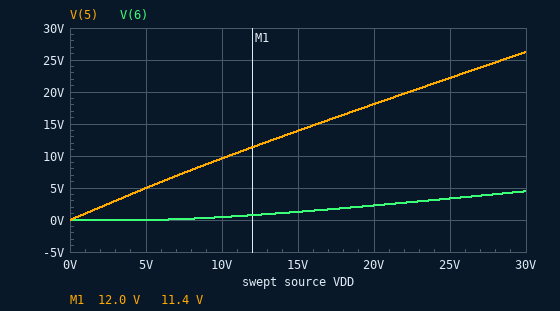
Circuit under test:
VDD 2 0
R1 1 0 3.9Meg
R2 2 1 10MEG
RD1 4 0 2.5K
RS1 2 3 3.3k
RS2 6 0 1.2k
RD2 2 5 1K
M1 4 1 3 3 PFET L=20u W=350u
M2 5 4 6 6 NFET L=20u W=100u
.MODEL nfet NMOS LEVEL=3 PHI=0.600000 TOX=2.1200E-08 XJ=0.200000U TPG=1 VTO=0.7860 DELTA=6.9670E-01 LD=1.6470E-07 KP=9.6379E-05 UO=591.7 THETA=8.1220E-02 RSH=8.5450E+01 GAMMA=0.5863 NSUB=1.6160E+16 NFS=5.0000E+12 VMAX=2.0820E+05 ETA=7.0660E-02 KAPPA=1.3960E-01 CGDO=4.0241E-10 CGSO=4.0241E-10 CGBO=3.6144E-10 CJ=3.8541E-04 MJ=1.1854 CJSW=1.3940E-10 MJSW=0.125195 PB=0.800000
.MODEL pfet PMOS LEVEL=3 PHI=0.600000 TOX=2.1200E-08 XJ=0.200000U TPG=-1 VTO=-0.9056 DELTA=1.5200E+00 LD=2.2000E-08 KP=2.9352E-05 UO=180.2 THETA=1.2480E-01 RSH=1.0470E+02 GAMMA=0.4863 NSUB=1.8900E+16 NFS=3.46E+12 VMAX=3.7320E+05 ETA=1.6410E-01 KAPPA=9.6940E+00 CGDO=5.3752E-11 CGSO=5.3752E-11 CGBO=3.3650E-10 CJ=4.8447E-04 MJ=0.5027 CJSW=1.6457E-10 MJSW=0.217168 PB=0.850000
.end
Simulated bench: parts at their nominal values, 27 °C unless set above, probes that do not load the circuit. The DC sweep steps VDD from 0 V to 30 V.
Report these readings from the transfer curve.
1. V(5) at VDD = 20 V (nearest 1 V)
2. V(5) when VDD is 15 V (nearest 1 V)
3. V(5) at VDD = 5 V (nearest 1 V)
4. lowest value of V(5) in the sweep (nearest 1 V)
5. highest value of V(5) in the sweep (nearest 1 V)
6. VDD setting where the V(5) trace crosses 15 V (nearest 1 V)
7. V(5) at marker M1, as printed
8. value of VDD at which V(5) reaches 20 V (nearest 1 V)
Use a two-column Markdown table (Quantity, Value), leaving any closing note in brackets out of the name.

| Quantity | Value |
|---|---|
| V(5) at VDD = 20 V | 18 V |
| V(5) when VDD is 15 V | 14 V |
| V(5) at VDD = 5 V | 5 V |
| lowest value of V(5) in the sweep | 0 V |
| highest value of V(5) in the sweep | 26 V |
| VDD setting where the V(5) trace crosses 15 V | 16 V |
| V(5) at marker M1, as printed | 11.4 V |
| value of VDD at which V(5) reaches 20 V | 22 V |
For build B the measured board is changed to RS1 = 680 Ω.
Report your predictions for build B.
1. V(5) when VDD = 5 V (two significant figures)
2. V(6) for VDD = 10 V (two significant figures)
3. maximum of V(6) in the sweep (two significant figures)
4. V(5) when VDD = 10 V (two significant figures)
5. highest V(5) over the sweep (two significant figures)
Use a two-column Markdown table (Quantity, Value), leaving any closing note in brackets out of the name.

| Quantity | Value |
|---|---|
| V(5) when VDD = 5 V | 4.8 V |
| V(6) for VDD = 10 V | 1.8 V |
| maximum of V(6) in the sweep | 9.8 V |
| V(5) when VDD = 10 V | 8.5 V |
| highest V(5) over the sweep | 22 V |
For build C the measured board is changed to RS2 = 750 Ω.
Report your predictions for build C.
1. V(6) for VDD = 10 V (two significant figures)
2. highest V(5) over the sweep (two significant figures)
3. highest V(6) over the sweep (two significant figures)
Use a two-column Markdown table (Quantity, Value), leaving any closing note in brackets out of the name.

| Quantity | Value |
|---|---|
| V(6) for VDD = 10 V | 330 mV |
| highest V(5) over the sweep | 25 V |
| highest V(6) over the sweep | 3.6 V |
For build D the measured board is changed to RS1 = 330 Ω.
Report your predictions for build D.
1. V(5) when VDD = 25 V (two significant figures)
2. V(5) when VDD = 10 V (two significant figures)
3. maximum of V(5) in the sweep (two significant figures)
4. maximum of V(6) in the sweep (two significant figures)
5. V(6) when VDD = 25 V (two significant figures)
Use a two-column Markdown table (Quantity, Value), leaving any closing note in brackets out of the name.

| Quantity | Value |
|---|---|
| V(5) when VDD = 25 V | 18 V |
| V(5) when VDD = 10 V | 8.2 V |
| maximum of V(5) in the sweep | 21 V |
| maximum of V(6) in the sweep | 11 V |
| V(6) when VDD = 25 V | 8.8 V |
